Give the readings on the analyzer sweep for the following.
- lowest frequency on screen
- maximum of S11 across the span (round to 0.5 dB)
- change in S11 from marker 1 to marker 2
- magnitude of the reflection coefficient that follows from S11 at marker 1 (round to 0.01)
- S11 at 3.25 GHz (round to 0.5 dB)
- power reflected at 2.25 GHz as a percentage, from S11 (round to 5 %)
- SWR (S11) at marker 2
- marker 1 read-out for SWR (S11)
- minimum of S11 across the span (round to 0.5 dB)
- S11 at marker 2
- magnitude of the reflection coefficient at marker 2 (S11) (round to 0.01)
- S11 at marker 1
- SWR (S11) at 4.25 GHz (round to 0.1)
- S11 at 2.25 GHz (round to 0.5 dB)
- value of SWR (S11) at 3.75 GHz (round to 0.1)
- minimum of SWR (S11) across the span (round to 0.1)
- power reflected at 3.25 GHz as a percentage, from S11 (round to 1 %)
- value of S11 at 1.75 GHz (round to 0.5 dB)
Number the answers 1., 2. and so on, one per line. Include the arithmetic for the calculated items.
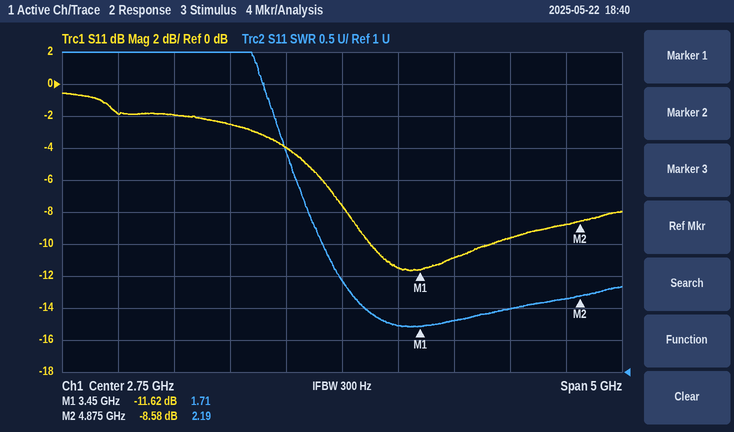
1. 250 MHz
2. -0.5 dB
3. -8.58 − (-11.62) = 3.04 dB
4. 10^(-11.62/20) ≈ 0.26
5. -11.5 dB
6. 10^(-4/10) ≈ 40 %
7. 2.19
8. 1.71
9. -11.5 dB
10. -8.58 dB
11. 10^(-8.58/20) ≈ 0.37
12. -11.62 dB
13. 2.0
14. -4.0 dB
15. 1.8
16. 1.7
17. 10^(-11.5/10) ≈ 7 %
18. -2.5 dB
